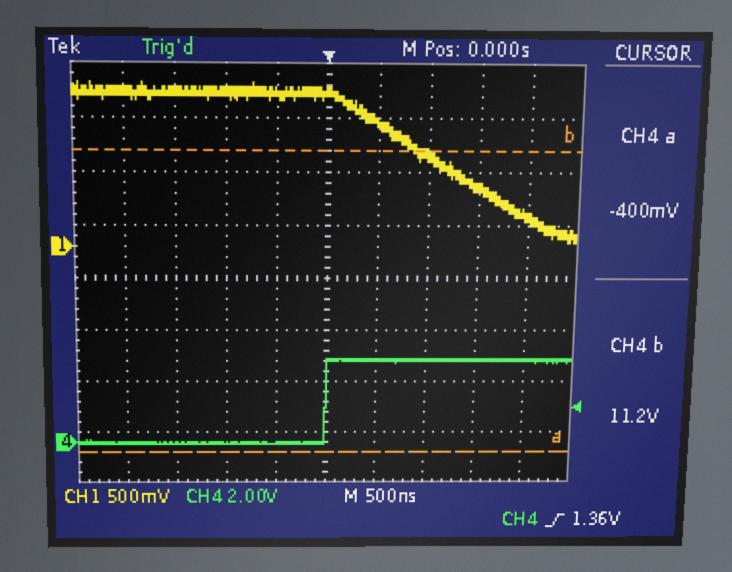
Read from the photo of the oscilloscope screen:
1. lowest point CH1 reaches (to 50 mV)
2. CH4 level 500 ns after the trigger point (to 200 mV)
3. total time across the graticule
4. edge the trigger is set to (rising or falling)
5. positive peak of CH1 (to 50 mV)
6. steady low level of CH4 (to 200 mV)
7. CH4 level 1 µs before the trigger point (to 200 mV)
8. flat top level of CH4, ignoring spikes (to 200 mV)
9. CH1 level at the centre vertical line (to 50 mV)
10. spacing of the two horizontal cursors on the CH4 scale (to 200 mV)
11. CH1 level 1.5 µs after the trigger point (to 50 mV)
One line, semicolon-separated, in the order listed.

50 mV; 3.2 V; 5 µs; rising; 1.50 V; 0.0 V; 0.0 V; 3.2 V; 1.45 V; 11.6 V; 550 mV
